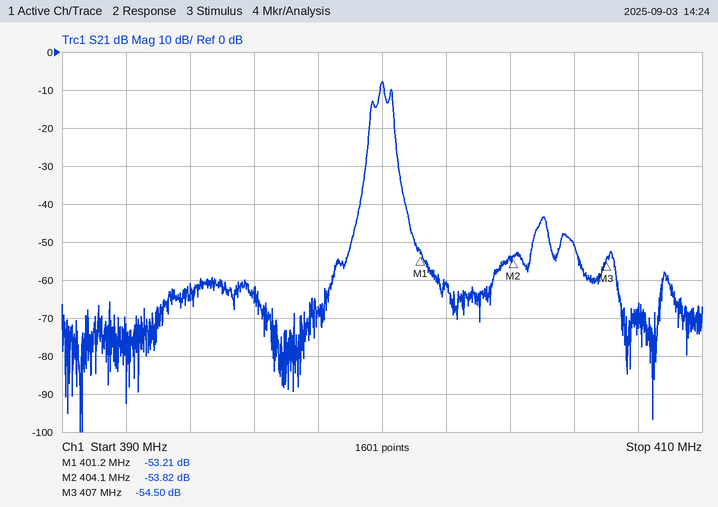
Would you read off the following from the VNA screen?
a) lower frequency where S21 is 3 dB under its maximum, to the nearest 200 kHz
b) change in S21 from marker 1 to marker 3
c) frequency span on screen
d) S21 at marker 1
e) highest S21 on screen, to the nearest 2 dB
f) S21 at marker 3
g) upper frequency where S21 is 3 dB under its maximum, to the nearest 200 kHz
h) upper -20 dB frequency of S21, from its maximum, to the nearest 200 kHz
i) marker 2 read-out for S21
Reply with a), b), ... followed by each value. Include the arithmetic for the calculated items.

a) 400.0 MHz
b) -54.5 − (-53.21) = -1.29 dB
c) 20 MHz
d) -53.21 dB
e) -8 dB
f) -54.50 dB
g) 400.0 MHz
h) 400.4 MHz
i) -53.82 dB
